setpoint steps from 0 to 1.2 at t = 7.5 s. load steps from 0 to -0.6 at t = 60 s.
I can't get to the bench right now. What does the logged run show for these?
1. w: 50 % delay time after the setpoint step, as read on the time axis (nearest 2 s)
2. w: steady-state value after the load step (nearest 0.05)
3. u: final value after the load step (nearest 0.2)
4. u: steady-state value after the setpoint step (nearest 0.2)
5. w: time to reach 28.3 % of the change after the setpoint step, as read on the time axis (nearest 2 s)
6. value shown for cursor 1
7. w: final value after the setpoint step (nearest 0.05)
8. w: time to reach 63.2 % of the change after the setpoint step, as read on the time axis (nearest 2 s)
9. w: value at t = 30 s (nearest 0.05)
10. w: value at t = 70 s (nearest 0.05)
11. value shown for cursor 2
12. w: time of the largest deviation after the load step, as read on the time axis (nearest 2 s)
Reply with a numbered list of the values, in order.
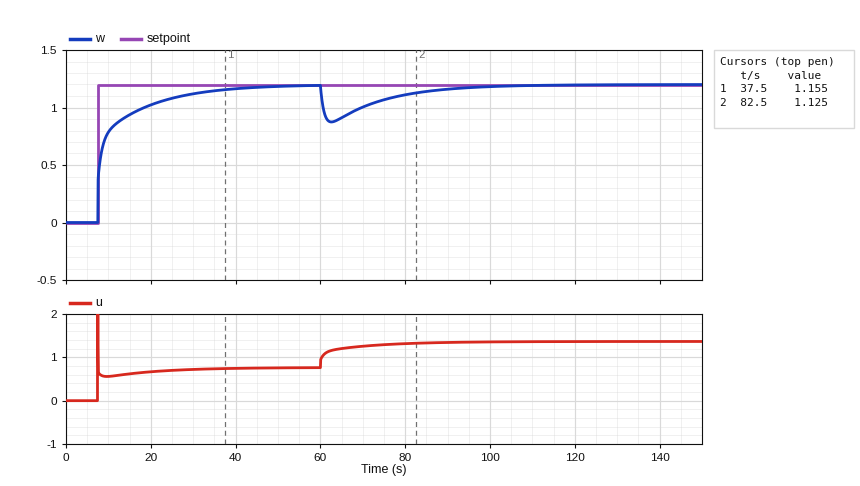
1. 8 s
2. 1.20
3. 1.4
4. 0.8
5. 8 s
6. 1.155
7. 1.20
8. 10 s
9. 1.10
10. 1.00
11. 1.125
12. 62 s
